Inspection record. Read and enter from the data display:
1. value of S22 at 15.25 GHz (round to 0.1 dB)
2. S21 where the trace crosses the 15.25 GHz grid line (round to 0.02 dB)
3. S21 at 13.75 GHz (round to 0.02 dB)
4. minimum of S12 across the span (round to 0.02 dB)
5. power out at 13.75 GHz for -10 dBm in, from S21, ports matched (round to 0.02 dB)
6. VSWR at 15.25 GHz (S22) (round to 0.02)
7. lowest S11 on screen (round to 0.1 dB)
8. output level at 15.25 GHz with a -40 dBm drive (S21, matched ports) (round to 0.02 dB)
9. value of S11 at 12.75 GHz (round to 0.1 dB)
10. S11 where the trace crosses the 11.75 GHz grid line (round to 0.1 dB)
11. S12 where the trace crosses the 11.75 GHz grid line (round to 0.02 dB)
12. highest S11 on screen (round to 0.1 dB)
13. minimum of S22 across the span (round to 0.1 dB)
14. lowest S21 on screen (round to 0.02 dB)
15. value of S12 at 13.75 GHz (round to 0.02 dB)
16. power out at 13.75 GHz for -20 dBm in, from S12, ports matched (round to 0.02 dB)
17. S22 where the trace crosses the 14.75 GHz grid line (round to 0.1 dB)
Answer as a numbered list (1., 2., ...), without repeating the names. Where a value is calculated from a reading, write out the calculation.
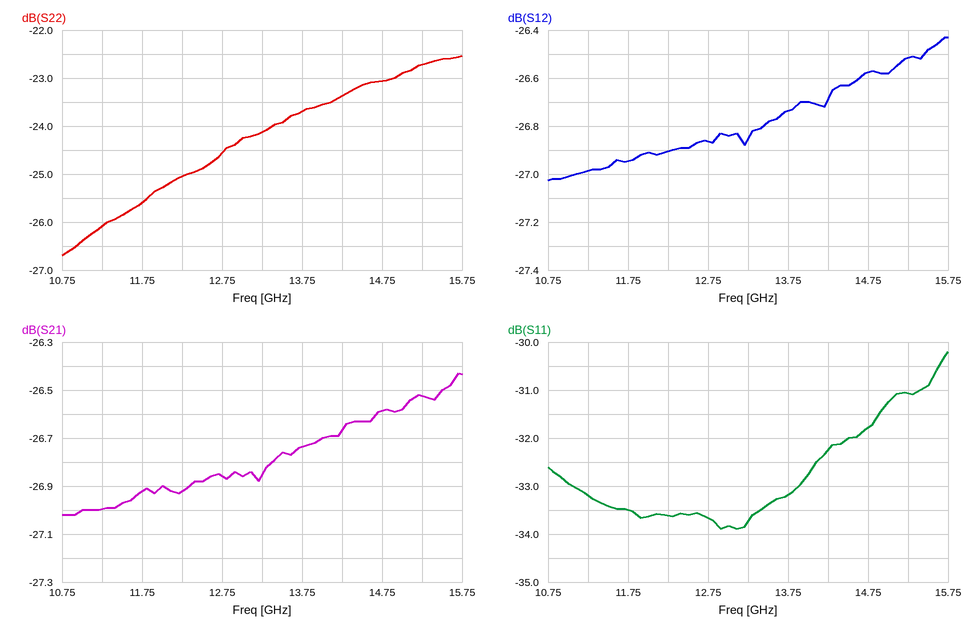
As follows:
1. -22.7 dB
2. -26.52 dB
3. -26.74 dB
4. -27.02 dB
5. -10 dBm + (-26.74 dB) = -36.74 dBm
6. |Γ| = 10^(-22.7/20) = 0.0733; VSWR = (1 + 0.0733)/(1 − 0.0733) ≈ 1.16
7. -33.9 dB
8. -40 dBm + (-26.52 dB) = -66.52 dBm
9. -33.7 dB
10. -33.5 dB
11. -26.94 dB
12. -30.2 dB
13. -26.7 dB
14. -27.02 dB
15. -26.74 dB
16. -20 dBm + (-26.74 dB) = -46.74 dBm
17. -23.1 dB
